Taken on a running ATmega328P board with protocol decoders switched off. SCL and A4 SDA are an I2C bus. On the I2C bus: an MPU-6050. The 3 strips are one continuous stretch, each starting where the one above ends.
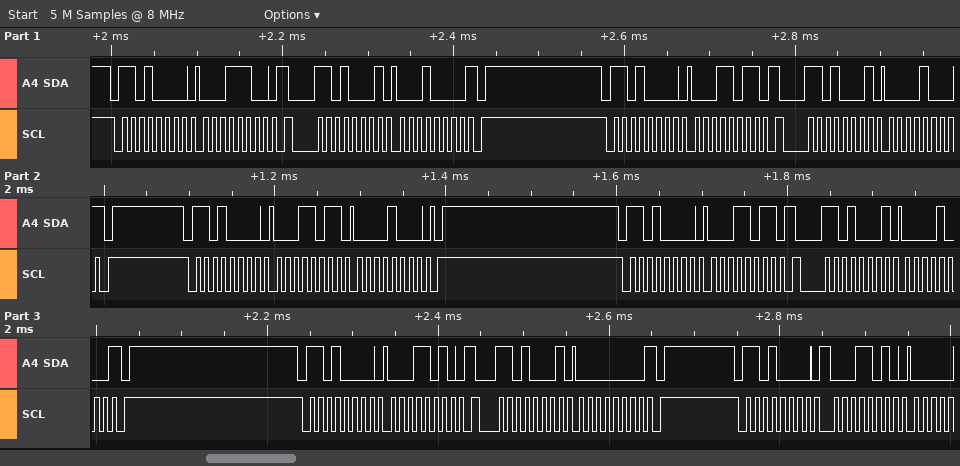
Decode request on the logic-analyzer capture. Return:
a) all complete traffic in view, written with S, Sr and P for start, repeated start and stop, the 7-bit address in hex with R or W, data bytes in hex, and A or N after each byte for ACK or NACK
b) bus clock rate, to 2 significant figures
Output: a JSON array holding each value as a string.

["S 68W A 1C A Sr 68R A 10 N P S 68W A 1B A Sr 68R A 08 N P S 68W A 1B A 08 A P S 68W A 1B A Sr 68R A 08 N P S 68W A 1A A Sr 68R A 00 N P S 68W A 1A A", "100 kHz"]
